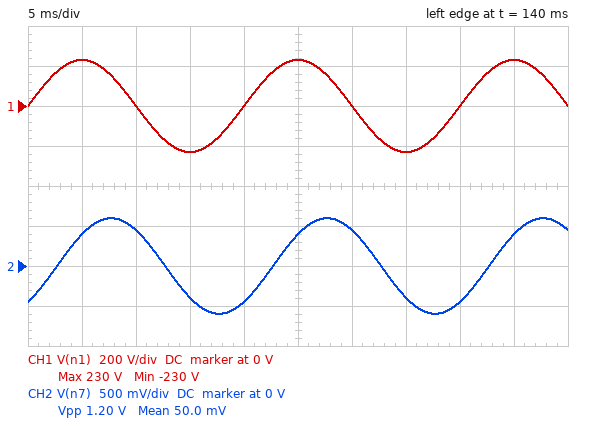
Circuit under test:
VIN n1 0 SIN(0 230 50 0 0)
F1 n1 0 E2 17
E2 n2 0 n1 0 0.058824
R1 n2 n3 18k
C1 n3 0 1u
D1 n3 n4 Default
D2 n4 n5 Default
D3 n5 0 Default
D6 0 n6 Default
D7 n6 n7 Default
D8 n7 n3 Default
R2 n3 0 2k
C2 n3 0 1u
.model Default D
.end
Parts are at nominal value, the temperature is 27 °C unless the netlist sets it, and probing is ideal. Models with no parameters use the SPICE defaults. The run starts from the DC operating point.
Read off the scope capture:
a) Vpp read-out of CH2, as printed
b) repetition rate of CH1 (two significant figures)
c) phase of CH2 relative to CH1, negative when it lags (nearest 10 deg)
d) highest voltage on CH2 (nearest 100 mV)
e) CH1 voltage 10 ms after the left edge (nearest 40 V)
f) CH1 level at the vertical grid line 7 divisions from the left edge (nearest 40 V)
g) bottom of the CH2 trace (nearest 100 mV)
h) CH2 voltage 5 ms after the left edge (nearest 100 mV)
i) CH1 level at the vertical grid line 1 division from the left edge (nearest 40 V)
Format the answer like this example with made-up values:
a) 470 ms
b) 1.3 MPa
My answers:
a) 1.20 V
b) 50 Hz
c) -50 deg
d) 600 mV
e) 0 V
f) -240 V
g) -600 mV
h) 400 mV
i) 240 V
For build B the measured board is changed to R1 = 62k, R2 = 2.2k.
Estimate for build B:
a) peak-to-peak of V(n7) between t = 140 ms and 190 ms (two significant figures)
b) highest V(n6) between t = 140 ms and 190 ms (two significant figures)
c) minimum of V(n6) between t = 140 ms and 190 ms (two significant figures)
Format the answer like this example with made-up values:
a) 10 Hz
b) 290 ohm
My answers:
a) 370 mV
b) 93 mV
c) -93 mV
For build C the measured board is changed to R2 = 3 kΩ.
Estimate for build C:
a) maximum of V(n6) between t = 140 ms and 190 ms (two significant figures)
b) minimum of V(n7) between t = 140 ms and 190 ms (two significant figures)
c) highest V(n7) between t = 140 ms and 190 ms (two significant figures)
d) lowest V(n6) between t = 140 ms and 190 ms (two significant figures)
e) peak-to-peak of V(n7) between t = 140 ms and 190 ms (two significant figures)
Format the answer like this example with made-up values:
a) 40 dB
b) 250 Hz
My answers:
a) 340 mV
b) -680 mV
c) 680 mV
d) -340 mV
e) 1.4 V
